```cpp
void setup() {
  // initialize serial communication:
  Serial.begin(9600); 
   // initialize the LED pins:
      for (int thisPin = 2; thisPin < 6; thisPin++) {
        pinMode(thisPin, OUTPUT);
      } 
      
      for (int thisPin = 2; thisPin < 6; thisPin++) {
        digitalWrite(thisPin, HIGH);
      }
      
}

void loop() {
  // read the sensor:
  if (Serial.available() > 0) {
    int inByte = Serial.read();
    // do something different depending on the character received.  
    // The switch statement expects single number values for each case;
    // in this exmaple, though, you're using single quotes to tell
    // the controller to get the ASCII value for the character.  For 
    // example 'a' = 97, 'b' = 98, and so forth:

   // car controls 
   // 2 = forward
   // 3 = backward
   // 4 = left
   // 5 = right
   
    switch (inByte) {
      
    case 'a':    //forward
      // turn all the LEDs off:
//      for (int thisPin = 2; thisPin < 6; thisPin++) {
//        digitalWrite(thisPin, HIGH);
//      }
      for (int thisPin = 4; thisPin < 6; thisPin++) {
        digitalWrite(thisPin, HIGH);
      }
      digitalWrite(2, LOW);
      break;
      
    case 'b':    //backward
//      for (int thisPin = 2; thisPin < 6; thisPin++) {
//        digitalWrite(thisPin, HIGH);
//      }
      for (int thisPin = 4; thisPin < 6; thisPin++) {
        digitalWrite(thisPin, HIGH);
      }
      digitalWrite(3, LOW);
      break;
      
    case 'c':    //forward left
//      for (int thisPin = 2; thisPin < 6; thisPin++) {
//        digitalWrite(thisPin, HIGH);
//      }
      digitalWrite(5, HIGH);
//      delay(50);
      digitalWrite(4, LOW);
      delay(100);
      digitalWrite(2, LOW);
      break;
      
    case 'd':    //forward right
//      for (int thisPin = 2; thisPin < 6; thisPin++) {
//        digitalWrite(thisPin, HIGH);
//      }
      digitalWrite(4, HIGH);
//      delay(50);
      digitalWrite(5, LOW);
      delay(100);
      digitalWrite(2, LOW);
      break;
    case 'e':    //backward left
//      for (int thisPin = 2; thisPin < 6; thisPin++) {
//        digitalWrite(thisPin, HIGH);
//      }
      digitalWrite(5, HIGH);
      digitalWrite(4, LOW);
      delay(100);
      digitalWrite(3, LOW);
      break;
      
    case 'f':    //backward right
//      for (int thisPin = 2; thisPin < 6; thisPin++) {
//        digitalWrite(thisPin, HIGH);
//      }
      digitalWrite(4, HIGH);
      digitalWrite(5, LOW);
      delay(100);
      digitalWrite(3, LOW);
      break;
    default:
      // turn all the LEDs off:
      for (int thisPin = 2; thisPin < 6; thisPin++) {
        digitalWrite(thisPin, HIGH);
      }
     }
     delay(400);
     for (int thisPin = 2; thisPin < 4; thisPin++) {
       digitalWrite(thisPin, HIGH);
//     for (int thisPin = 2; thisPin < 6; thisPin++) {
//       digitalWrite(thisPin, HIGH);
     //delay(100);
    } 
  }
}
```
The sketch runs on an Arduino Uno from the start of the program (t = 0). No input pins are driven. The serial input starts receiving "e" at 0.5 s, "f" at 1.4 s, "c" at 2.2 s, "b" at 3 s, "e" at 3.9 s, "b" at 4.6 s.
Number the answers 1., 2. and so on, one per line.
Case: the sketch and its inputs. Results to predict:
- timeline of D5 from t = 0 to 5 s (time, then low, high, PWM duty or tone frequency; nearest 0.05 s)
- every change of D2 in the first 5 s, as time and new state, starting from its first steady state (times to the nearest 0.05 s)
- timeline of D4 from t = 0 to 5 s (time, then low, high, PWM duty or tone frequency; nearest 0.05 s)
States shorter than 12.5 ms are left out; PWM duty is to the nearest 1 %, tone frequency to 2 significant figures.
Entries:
1. 0 s high; 1.4 s low; 2.2 s high
2. 0 s high; 2.3 s low; 2.7 s high
3. 0 s high; 0.5 s low; 1.4 s high; 2.2 s low; 3 s high; 3.9 s low; 4.6 s high
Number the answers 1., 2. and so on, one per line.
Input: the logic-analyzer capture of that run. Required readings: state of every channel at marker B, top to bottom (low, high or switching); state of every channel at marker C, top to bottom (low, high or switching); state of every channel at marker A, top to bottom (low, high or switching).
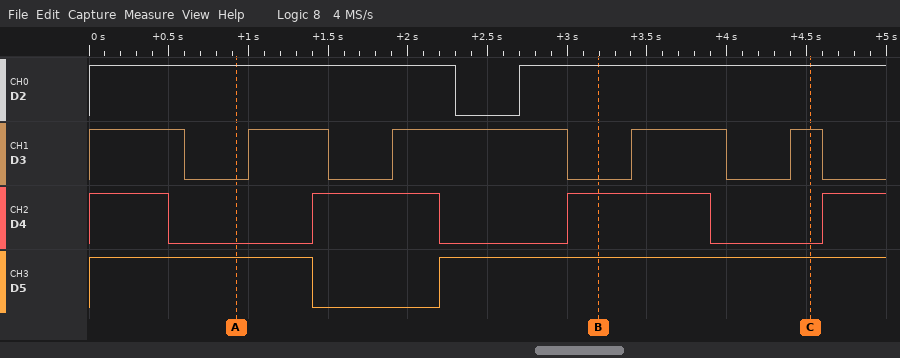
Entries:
1. D2 high, D3 low, D4 high, D5 high
2. D2 high, D3 high, D4 low, D5 high
3. D2 high, D3 low, D4 low, D5 high
